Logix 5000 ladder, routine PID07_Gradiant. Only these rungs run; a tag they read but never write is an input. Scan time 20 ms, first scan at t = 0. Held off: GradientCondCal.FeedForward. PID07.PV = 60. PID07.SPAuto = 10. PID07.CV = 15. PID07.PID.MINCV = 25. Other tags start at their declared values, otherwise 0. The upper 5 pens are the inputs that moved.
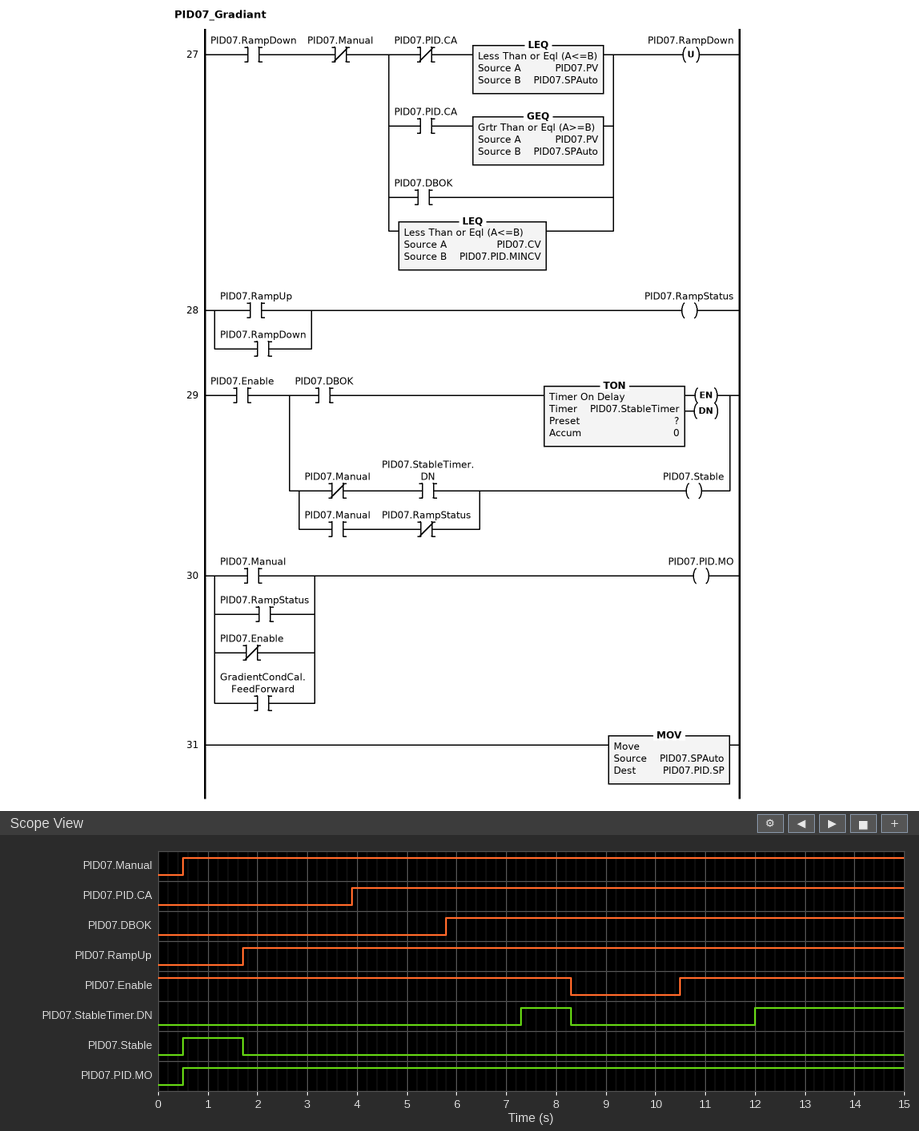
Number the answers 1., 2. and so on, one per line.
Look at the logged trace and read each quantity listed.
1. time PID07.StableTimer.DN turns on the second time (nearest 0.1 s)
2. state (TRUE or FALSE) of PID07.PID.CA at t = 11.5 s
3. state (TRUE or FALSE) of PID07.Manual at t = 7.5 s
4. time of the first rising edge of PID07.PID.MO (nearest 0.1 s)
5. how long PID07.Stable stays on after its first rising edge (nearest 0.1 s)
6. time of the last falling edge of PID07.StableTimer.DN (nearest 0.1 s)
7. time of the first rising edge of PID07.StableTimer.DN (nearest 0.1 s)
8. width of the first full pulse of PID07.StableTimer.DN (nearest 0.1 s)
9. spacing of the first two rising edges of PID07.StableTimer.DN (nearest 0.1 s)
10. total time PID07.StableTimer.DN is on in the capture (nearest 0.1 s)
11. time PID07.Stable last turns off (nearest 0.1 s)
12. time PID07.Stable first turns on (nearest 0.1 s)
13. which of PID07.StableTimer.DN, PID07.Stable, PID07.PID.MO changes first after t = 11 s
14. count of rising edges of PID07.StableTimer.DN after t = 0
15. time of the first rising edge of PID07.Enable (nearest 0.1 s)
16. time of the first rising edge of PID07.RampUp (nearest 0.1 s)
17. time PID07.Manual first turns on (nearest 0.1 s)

1. 12.0 s
2. TRUE
3. TRUE
4. 0.5 s
5. 1.2 s
6. 8.3 s
7. 7.3 s
8. 1.0 s
9. 4.7 s
10. 4.0 s
11. 1.7 s
12. 0.5 s
13. PID07.StableTimer.DN
14. 2
15. 10.5 s
16. 1.7 s
17. 0.5 s
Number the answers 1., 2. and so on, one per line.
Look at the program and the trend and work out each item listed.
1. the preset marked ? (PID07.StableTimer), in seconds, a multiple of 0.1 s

1. 1.5 s
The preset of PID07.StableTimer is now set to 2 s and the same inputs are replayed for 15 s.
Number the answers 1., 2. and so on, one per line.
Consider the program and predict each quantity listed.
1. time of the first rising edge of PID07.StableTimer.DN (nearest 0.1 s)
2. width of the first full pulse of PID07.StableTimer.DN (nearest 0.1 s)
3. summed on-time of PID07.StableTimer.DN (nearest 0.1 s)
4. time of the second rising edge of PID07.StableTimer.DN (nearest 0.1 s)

1. 7.8 s
2. 0.5 s
3. 3.0 s
4. 12.5 s
